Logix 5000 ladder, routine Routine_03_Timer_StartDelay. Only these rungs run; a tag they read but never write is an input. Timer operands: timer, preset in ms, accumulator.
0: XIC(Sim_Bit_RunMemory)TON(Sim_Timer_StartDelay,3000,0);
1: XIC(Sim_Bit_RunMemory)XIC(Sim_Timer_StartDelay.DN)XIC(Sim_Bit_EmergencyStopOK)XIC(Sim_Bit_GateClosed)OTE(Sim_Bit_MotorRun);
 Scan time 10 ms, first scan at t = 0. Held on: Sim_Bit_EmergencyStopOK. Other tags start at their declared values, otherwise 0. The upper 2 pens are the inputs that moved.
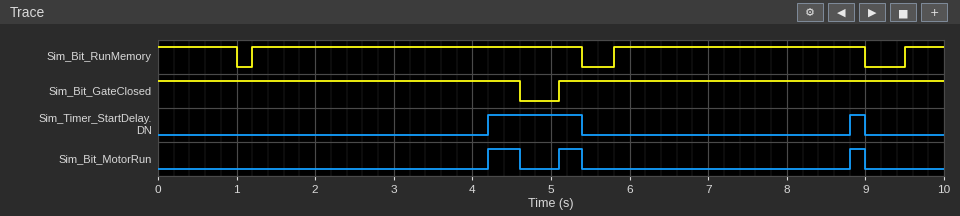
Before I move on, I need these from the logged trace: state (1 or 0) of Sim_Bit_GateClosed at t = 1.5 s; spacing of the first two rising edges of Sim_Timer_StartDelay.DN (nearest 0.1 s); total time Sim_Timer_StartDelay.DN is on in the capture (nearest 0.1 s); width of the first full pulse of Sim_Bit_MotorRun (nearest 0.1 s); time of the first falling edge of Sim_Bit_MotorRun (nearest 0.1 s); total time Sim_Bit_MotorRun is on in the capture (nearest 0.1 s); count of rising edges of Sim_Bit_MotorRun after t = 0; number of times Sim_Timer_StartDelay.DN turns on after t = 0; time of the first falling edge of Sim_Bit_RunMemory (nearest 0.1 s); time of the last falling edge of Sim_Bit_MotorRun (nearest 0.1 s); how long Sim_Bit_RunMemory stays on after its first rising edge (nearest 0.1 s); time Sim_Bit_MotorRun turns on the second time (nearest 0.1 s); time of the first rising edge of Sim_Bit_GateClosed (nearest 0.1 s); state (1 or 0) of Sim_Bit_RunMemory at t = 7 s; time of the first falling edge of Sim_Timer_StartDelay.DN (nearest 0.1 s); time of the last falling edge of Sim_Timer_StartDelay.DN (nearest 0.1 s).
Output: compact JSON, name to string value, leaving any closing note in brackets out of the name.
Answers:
{"state (1 or 0) of Sim_Bit_GateClosed at t = 1.5 s": "1", "spacing of the first two rising edges of Sim_Timer_StartDelay.DN": "4.6 s", "total time Sim_Timer_StartDelay.DN is on in the capture": "1.4 s", "width of the first full pulse of Sim_Bit_MotorRun": "0.4 s", "time of the first falling edge of Sim_Bit_MotorRun": "4.6 s", "total time Sim_Bit_MotorRun is on in the capture": "0.9 s", "count of rising edges of Sim_Bit_MotorRun after t = 0": "3", "number of times Sim_Timer_StartDelay.DN turns on after t = 0": "2", "time of the first falling edge of Sim_Bit_RunMemory": "1.0 s", "time of the last falling edge of Sim_Bit_MotorRun": "9.0 s", "how long Sim_Bit_RunMemory stays on after its first rising edge": "4.2 s", "time Sim_Bit_MotorRun turns on the second time": "5.1 s", "time of the first rising edge of Sim_Bit_GateClosed": "5.1 s", "state (1 or 0) of Sim_Bit_RunMemory at t = 7 s": "1", "time of the first falling edge of Sim_Timer_StartDelay.DN": "5.4 s", "time of the last falling edge of Sim_Timer_StartDelay.DN": "9.0 s"}
